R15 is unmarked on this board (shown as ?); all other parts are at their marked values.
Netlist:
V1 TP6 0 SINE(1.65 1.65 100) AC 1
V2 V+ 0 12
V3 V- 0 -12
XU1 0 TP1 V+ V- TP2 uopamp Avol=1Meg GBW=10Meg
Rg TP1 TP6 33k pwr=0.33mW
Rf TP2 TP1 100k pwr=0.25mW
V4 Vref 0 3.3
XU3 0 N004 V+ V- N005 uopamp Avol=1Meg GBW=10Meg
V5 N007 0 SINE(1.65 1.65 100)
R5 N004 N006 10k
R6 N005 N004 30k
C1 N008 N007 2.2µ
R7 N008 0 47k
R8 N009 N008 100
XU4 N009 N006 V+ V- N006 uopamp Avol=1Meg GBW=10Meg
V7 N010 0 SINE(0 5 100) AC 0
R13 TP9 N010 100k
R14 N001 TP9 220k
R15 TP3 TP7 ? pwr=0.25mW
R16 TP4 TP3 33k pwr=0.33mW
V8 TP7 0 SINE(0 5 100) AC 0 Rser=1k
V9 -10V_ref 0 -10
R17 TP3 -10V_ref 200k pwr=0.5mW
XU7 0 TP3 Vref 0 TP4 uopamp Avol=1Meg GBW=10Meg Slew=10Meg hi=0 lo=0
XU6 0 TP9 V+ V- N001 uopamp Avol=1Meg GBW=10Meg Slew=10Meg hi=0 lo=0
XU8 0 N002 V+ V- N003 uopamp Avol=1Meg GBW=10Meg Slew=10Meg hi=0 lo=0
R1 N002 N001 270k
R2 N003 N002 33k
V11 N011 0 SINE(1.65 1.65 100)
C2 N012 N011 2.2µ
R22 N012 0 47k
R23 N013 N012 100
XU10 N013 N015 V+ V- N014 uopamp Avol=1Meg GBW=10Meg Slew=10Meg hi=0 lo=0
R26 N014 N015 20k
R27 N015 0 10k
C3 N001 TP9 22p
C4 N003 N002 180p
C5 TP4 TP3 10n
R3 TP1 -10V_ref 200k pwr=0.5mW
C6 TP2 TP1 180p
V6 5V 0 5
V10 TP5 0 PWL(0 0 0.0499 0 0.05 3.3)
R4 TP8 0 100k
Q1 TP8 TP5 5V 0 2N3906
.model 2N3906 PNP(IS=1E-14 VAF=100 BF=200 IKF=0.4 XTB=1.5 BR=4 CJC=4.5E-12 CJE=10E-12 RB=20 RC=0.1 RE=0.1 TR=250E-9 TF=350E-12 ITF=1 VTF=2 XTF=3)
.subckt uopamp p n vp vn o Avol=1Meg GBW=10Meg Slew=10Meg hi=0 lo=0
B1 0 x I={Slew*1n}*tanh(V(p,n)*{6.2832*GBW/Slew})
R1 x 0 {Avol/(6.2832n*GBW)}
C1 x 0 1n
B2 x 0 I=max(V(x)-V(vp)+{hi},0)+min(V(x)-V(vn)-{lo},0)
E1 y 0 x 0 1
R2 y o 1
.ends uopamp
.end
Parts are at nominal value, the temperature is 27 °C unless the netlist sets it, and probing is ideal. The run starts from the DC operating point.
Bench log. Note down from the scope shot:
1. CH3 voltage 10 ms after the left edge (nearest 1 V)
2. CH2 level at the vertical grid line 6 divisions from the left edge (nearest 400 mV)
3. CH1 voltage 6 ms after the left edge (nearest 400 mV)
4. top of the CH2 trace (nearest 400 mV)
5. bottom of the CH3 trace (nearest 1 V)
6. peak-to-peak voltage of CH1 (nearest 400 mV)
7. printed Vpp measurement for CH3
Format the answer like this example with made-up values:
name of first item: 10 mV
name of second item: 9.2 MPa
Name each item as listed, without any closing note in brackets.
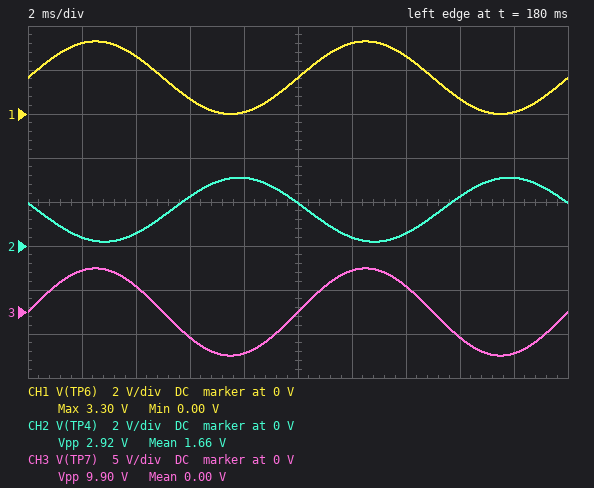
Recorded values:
CH3 voltage 10 ms after the left edge: 0 V
CH2 level at the vertical grid line 6 divisions from the left edge: 400 mV
CH1 voltage 6 ms after the left edge: 800 mV
top of the CH2 trace: 3.2 V
bottom of the CH3 trace: -5 V
peak-to-peak voltage of CH1: 3.2 V
printed Vpp measurement for CH3: 9.90 V
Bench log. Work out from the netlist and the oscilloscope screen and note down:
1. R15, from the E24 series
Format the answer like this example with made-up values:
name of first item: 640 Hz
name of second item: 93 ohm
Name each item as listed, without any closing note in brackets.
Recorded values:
R15, from the E24 series: 110 kΩ
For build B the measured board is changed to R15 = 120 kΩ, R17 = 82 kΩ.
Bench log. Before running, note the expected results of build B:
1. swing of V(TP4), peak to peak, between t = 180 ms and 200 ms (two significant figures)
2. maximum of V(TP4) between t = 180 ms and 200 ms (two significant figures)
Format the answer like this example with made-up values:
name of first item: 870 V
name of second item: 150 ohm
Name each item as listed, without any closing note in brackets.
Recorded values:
swing of V(TP4), peak to peak, between t = 180 ms and 200 ms: 620 mV
maximum of V(TP4) between t = 180 ms and 200 ms: 3.3 V
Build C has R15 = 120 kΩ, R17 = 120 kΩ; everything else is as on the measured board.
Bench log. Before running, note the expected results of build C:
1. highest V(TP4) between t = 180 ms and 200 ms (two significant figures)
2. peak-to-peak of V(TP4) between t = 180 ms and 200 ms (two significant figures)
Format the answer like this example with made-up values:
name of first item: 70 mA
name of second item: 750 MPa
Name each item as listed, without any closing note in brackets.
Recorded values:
highest V(TP4) between t = 180 ms and 200 ms: 3.3 V
peak-to-peak of V(TP4) between t = 180 ms and 200 ms: 1.9 V
